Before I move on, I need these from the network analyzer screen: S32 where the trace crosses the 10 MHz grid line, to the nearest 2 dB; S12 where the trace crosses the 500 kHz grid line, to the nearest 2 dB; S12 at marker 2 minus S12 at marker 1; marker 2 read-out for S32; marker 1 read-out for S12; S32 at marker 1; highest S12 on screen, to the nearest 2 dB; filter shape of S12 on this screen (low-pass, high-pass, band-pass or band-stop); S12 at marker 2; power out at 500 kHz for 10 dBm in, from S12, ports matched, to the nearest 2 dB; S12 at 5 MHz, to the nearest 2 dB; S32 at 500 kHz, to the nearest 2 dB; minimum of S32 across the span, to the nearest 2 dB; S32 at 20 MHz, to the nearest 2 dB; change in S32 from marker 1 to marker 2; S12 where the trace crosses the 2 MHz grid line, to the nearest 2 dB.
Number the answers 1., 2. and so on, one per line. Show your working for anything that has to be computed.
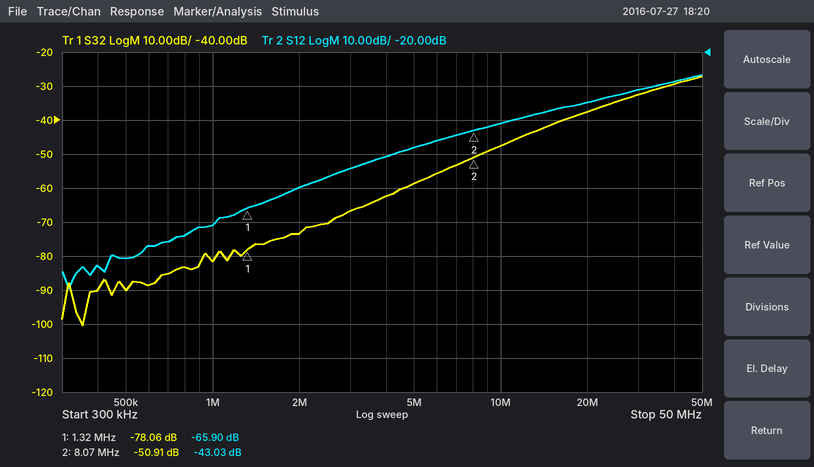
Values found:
1. -48 dB
2. -80 dB
3. -43.03 − (-65.9) = 22.87 dB
4. -50.91 dB
5. -65.90 dB
6. -78.06 dB
7. -26 dB
8. high-pass
9. -43.03 dB
10. 10 dBm + (-80 dB) = -70 dBm
11. -48 dB
12. -90 dB
13. -100 dB
14. -38 dB
15. -50.91 − (-78.06) = 27.15 dB
16. -60 dB
